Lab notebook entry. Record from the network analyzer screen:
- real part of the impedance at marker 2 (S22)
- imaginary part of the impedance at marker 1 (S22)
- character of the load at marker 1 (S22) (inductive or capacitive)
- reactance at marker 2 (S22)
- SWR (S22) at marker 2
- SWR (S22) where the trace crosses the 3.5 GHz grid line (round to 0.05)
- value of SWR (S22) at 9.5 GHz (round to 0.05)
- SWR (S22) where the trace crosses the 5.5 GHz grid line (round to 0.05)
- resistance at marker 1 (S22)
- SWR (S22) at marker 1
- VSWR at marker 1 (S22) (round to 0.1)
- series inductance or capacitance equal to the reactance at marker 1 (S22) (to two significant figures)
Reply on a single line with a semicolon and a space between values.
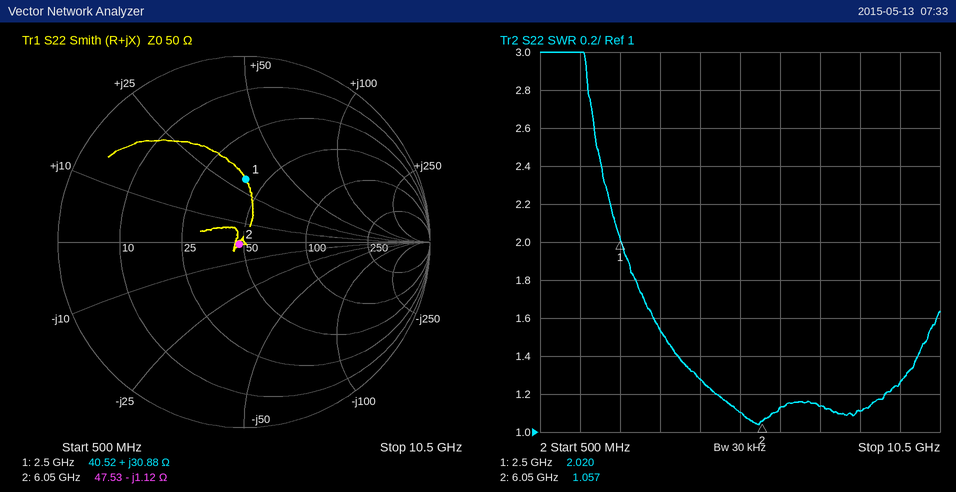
47.53 Ω; +30.88 Ω; inductive; -1.12 Ω; 1.057; 1.55; 1.25; 1.10; 40.52 Ω; 2.020; 2.0; 2.0 nH
